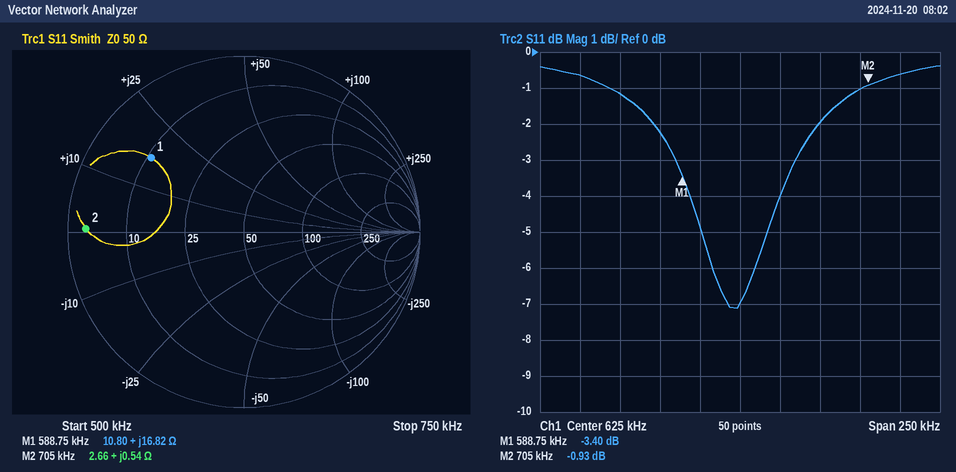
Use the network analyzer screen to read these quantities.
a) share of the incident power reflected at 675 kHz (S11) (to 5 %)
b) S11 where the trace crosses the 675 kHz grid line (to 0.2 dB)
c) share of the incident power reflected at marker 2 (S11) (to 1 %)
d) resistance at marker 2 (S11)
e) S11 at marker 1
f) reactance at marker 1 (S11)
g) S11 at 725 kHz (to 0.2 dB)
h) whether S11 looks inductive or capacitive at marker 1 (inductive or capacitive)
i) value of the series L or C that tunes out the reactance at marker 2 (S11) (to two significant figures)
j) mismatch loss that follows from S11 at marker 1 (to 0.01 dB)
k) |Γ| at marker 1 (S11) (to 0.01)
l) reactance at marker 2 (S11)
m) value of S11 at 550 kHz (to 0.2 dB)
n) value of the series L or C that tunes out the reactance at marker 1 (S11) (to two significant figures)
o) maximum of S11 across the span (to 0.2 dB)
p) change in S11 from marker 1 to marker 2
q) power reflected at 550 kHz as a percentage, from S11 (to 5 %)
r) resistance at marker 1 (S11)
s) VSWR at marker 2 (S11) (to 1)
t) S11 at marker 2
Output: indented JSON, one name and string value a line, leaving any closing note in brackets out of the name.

{
  "share of the incident power reflected at 675 kHz (S11)": "65 %",
  "S11 where the trace crosses the 675 kHz grid line": "-2.0 dB",
  "share of the incident power reflected at marker 2 (S11)": "81 %",
  "resistance at marker 2": "2.66 Ω",
  "S11 at marker 1": "-3.40 dB",
  "reactance at marker 1": "+16.82 Ω",
  "S11 at 725 kHz": "-0.6 dB",
  "whether S11 looks inductive or capacitive at marker 1": "inductive",
  "value of the series L or C that tunes out the reactance at marker 2 (S11)": "420 nF",
  "mismatch loss that follows from S11 at marker 1": "2.65 dB",
  "|Γ| at marker 1 (S11)": "0.68",
  "reactance at marker 2": "+0.54 Ω",
  "value of S11 at 550 kHz": "-1.2 dB",
  "value of the series L or C that tunes out the reactance at marker 1 (S11)": "16 nF",
  "maximum of S11 across the span": "-0.4 dB",
  "change in S11 from marker 1 to marker 2": "2.47 dB",
  "power reflected at 550 kHz as a percentage, from S11": "75 %",
  "resistance at marker 1": "10.80 Ω",
  "VSWR at marker 2 (S11)": "19",
  "S11 at marker 2": "-0.93 dB"
}
